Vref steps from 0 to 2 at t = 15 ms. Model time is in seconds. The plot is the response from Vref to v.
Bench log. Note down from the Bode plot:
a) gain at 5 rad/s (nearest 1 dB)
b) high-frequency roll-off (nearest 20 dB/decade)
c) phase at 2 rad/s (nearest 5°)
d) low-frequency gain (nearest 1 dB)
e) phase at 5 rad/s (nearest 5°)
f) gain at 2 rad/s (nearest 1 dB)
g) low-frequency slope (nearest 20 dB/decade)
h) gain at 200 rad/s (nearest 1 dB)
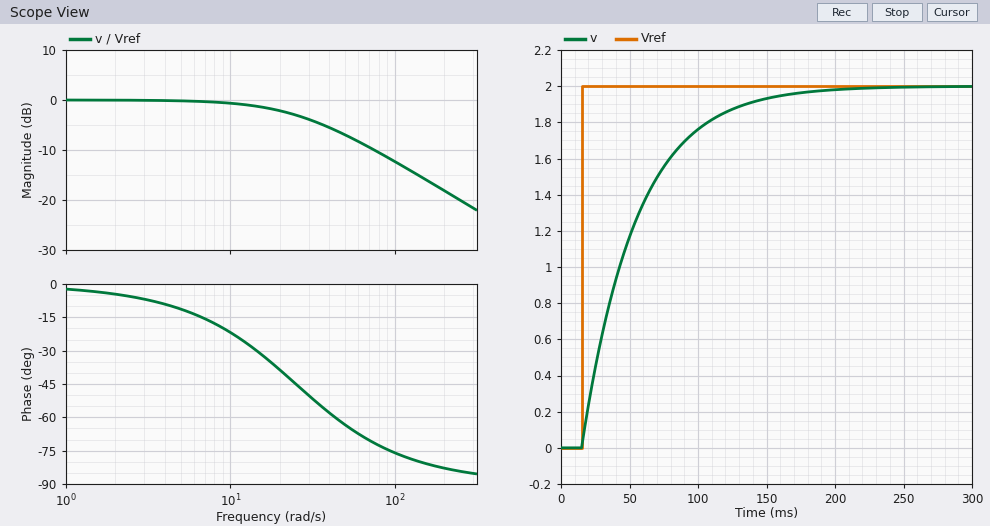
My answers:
0 dB
-20 dB/decade
-5°
0 dB
-10°
0 dB
0 dB/decade
-18 dB
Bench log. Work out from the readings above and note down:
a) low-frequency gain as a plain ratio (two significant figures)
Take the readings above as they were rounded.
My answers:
1.0
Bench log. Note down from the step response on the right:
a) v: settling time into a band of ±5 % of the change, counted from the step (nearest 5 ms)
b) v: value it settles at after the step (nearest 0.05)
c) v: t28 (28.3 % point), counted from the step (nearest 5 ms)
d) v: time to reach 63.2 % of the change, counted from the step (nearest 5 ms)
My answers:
120 ms
2.00
15 ms
40 ms
